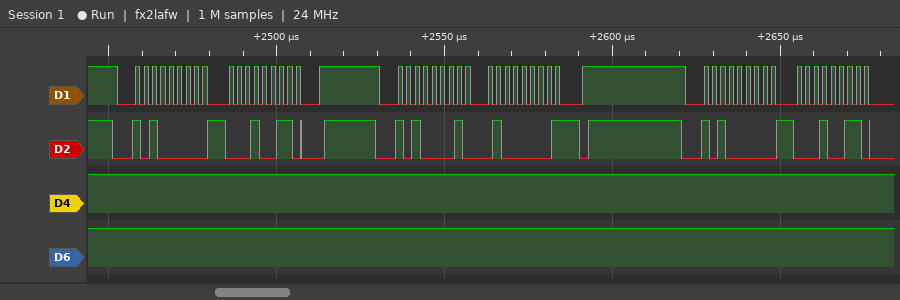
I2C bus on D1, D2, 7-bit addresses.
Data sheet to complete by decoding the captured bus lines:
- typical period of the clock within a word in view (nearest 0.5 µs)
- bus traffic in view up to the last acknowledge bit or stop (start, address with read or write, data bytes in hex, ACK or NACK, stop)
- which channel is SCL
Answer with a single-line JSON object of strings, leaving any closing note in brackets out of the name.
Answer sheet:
{"typical period of the clock within a word in view": "2.5 µs", "bus traffic in view up to the last acknowledge bit or stop": "start, address 50 write ACK, 13 ACK, stop, start, address 50 read ACK, 40 NACK, stop, start, address 50 write ACK, 13 ACK", "which channel is SCL": "D1"}
